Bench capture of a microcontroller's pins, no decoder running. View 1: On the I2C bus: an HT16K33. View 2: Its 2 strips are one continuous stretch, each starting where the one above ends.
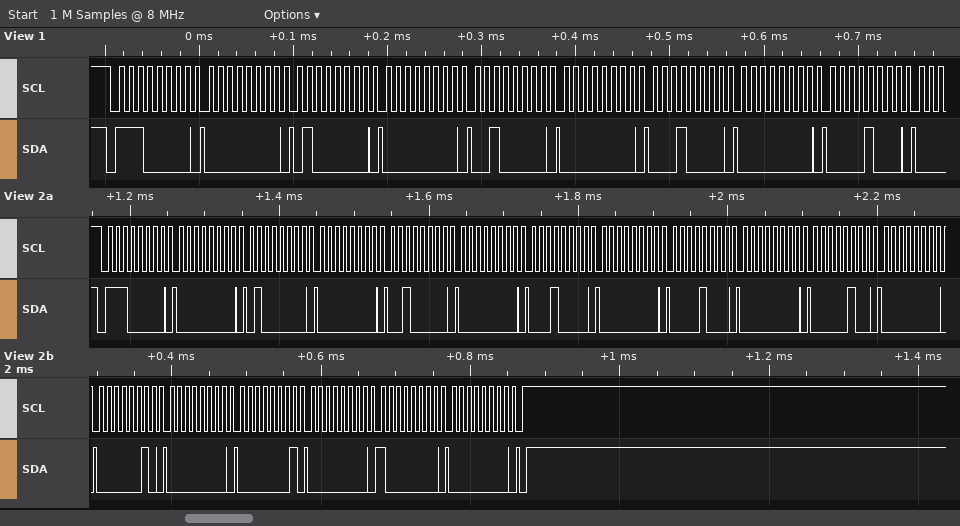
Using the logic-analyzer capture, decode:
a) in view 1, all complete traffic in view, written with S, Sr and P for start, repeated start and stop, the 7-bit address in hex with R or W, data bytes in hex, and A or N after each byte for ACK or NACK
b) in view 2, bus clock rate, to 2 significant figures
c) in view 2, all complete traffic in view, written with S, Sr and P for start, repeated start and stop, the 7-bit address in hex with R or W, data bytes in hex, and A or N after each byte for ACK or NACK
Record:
S 70W A 00 A 40 A 00 A 20 A 00 A 10 A 00 A 08 A
100 kHz
S 70W A 00 A 40 A 00 A 20 A 00 A 10 A 00 A 08 A 00 A 04 A 00 A 02 A 00 A 01 A 00 A 80 A 00 A P
